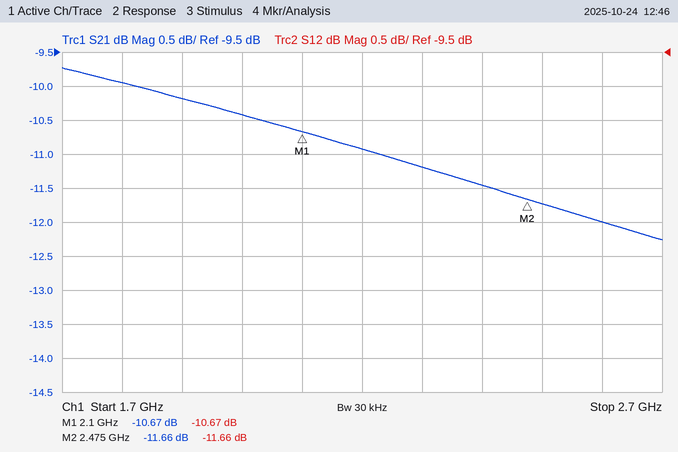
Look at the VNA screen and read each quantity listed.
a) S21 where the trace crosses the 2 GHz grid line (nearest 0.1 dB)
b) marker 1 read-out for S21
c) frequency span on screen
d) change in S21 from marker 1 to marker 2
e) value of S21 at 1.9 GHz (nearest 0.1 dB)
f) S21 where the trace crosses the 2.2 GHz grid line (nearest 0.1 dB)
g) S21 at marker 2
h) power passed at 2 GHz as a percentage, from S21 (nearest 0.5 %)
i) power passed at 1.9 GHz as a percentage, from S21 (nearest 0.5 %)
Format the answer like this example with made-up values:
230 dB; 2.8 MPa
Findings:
-10.4 dB; -10.67 dB; 1 GHz; -0.99 dB; -10.2 dB; -10.9 dB; -11.66 dB; 9.0 %; 9.5 %
